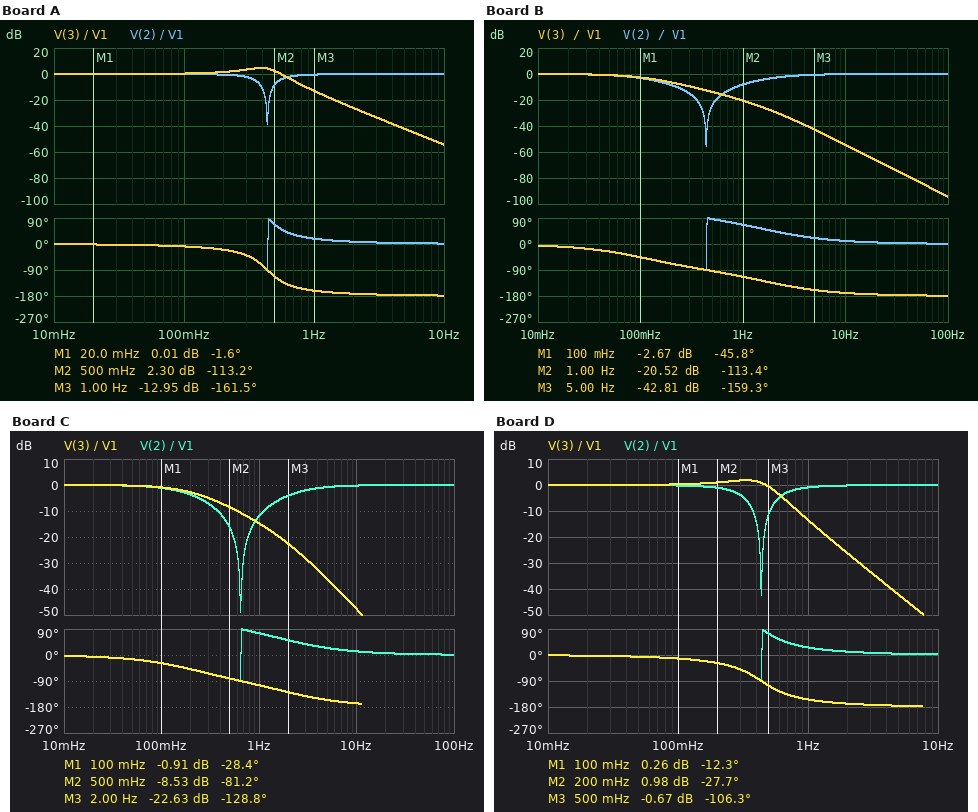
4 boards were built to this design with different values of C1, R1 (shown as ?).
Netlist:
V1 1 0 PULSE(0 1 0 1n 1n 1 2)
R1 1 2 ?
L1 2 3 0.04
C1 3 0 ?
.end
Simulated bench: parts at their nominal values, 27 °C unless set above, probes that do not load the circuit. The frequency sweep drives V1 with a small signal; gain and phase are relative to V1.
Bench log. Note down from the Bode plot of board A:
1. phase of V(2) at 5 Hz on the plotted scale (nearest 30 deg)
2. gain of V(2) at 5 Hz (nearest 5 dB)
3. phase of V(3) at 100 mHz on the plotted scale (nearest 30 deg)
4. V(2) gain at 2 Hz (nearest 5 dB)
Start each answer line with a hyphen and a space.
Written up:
- 0 deg
- 0 dB
- 0 deg
- 0 dB
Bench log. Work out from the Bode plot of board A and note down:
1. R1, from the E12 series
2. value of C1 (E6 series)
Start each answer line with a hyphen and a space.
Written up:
- 0.068 Ω
- 3.3 F
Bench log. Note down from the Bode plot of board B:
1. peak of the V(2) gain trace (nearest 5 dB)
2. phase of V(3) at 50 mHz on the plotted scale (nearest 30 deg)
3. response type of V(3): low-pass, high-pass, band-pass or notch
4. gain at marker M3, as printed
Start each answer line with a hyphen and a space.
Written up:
- 0 dB
- -30 deg
- low-pass
- -42.81 dB
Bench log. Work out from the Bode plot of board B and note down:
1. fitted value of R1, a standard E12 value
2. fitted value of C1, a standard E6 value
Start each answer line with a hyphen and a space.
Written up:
- 0.47 Ω
- 3.3 F
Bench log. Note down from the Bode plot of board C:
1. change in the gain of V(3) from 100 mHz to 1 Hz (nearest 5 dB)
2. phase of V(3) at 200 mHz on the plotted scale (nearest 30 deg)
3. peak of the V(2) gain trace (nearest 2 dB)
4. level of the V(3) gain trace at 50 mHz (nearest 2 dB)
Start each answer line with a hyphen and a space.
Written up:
- -15 dB
- -60 deg
- 0 dB
- 0 dB
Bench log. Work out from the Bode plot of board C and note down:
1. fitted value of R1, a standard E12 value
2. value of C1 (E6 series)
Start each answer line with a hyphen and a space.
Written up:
- 0.56 Ω
- 1.5 F
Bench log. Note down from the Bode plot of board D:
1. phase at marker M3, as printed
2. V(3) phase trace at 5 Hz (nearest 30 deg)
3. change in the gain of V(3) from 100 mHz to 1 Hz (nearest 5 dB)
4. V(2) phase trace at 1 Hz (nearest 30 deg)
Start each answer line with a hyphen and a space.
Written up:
- -106.3 deg
- -180 deg
- -15 dB
- 30 deg
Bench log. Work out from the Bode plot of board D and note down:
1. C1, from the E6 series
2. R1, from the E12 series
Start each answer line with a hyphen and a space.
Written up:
- 3.3 F
- 0.1 Ω
